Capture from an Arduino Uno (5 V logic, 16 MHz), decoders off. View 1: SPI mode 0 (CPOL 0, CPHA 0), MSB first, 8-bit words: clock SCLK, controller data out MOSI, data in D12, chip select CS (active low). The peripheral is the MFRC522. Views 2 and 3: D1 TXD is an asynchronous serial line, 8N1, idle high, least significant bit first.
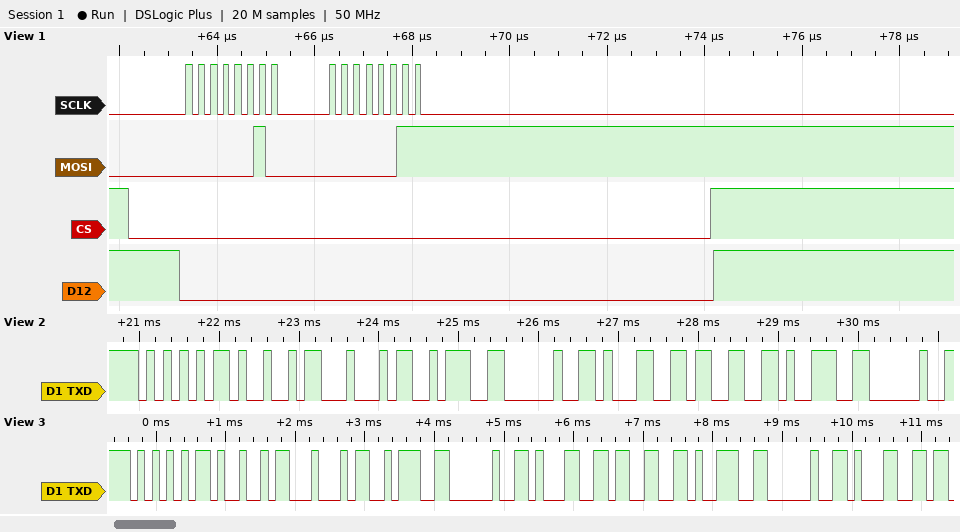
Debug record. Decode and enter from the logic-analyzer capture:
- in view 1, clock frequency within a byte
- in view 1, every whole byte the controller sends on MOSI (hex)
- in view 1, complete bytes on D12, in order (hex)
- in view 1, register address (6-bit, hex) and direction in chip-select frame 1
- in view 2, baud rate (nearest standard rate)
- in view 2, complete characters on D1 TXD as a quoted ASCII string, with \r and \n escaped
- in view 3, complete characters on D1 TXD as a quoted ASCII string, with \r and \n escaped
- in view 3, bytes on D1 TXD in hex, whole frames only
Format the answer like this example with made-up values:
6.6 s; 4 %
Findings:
4 MHz; 02 03; 00 00; 0x01 write; 9600 baud; "UID: 139 "; "UID: 139 1"; 55 49 44 3A 20 31 33 39 20 31
